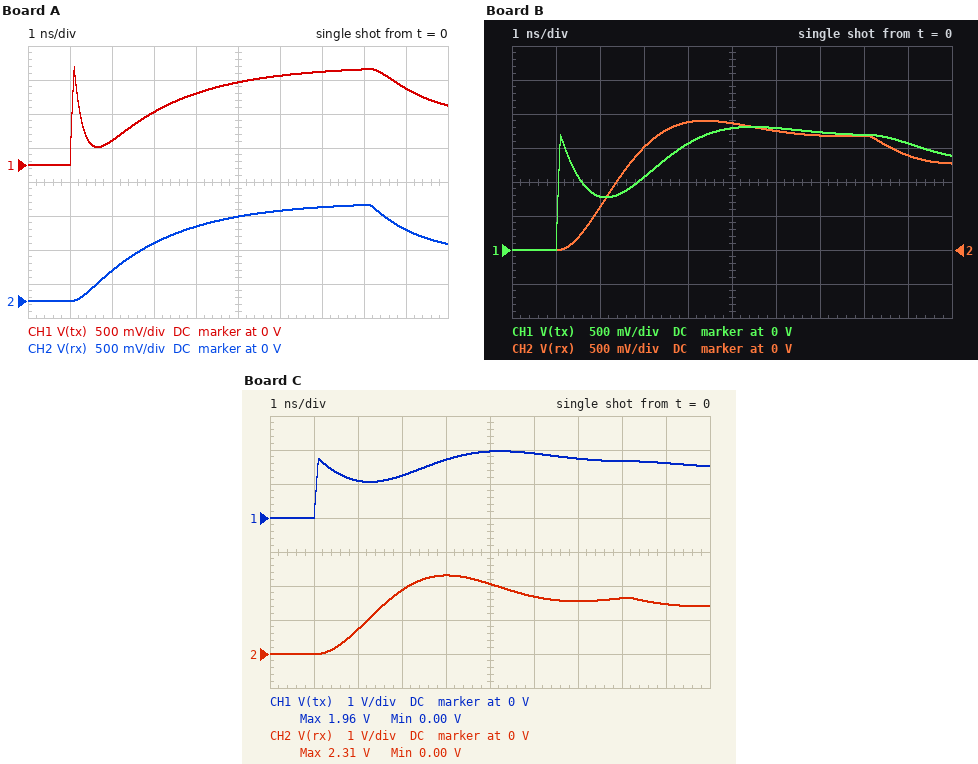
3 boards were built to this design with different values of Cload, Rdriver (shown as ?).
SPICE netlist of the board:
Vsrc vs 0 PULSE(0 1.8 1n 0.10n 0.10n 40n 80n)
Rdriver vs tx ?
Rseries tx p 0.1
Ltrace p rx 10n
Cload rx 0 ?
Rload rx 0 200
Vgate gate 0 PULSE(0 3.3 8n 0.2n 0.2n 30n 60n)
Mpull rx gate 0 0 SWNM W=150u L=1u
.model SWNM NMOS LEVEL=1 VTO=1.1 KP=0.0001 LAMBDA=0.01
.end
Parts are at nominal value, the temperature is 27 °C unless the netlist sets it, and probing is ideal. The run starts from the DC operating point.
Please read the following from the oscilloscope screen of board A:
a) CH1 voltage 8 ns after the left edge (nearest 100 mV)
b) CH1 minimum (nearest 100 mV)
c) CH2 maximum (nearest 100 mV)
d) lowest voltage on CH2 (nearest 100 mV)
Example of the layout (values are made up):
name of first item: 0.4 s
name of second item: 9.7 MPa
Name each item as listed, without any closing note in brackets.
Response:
CH1 voltage 8 ns after the left edge: 1.4 V
CH1 minimum: 0 V
CH2 maximum: 1.4 V
lowest voltage on CH2: 0 V
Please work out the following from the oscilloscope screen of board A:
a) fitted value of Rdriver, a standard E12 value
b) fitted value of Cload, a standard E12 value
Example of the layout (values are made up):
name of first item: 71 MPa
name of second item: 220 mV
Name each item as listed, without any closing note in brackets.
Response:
fitted value of Rdriver, a standard E12 value: 47 Ω
fitted value of Cload, a standard E12 value: 56 pF
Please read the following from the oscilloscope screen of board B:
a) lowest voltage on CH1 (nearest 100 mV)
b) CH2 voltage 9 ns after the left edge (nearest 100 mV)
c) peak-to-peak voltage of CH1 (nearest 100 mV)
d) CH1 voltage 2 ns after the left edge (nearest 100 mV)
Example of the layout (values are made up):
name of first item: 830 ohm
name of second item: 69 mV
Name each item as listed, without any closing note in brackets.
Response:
lowest voltage on CH1: 0 V
CH2 voltage 9 ns after the left edge: 1.4 V
peak-to-peak voltage of CH1: 1.8 V
CH1 voltage 2 ns after the left edge: 800 mV
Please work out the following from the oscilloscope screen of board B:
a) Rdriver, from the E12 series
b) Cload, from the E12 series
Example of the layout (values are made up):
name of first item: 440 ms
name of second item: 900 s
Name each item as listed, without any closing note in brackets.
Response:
Rdriver, from the E12 series: 12 Ω
Cload, from the E12 series: 82 pF
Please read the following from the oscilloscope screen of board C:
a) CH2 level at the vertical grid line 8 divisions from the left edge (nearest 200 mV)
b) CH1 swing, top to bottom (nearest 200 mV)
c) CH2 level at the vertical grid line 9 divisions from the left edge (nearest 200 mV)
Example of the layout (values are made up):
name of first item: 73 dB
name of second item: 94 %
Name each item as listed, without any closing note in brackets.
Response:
CH2 level at the vertical grid line 8 divisions from the left edge: 1.6 V
CH1 swing, top to bottom: 2.0 V
CH2 level at the vertical grid line 9 divisions from the left edge: 1.4 V
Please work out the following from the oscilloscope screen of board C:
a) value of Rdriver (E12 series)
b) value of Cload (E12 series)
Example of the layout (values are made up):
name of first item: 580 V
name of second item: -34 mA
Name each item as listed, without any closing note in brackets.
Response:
value of Rdriver: 6.8 Ω
value of Cload: 82 pF
